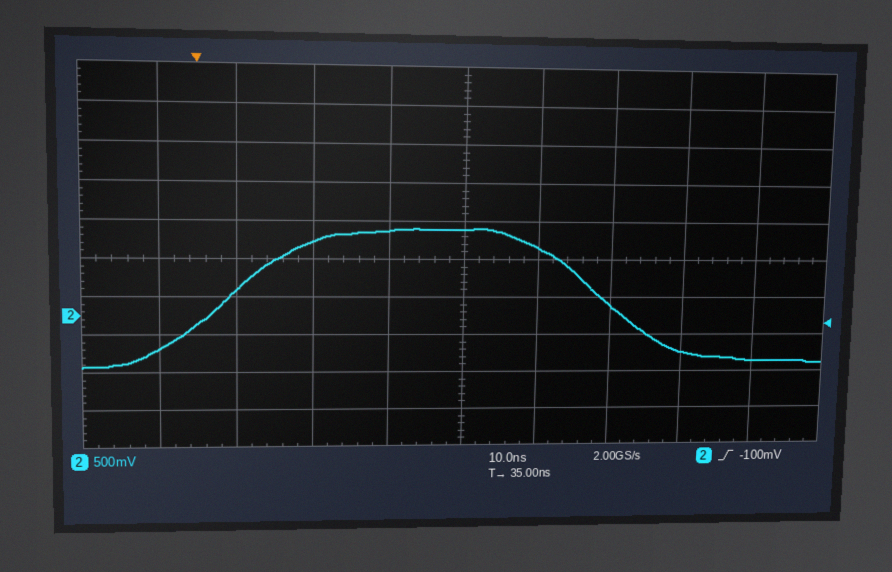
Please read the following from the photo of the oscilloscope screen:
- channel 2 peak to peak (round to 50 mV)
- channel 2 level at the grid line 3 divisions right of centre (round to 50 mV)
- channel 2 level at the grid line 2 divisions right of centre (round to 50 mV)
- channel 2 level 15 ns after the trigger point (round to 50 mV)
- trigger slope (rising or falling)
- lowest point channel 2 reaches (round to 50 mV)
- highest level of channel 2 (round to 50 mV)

1.85 V
-500 mV
150 mV
1.00 V
rising
-700 mV
1.15 V
